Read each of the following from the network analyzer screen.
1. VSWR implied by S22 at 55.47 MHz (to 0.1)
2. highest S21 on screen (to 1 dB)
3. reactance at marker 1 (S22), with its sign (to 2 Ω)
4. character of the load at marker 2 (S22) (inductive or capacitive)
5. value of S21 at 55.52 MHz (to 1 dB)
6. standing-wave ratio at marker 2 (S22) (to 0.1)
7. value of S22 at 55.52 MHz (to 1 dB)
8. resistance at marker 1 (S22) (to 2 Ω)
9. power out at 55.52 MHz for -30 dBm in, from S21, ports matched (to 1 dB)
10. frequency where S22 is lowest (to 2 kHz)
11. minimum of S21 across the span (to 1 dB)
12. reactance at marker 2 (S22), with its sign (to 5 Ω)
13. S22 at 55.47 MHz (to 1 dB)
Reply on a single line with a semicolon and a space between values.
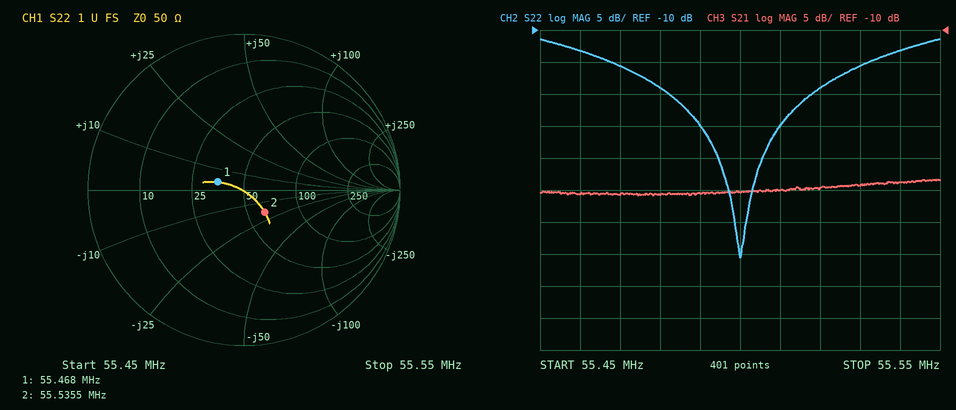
1.4; -33 dB; +4 Ω; capacitive; -35 dB; 1.5; -19 dB; 36 Ω; -65 dBm; 55.500 MHz; -36 dB; -20 Ω; -16 dB
